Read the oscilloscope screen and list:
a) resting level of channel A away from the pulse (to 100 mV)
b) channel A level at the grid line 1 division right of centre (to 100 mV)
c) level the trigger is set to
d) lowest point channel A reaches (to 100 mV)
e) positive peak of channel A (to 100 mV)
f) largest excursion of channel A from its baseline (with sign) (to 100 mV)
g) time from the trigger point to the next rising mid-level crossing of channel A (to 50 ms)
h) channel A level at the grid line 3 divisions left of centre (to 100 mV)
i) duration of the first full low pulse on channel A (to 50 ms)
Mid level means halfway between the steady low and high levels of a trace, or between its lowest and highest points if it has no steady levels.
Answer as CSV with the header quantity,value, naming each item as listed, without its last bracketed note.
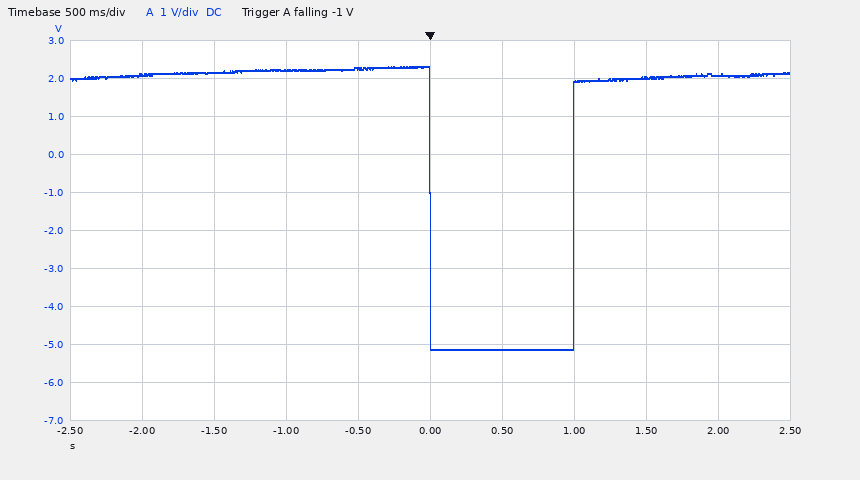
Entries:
quantity,value
resting level of channel A away from the pulse,2.1 V
channel A level at the grid line 1 division right of centre,-5.1 V
level the trigger is set to,-1 V
lowest point channel A reaches,-5.1 V
positive peak of channel A,2.3 V
largest excursion of channel A from its baseline (with sign),-7.2 V
time from the trigger point to the next rising mid-level crossing of channel A,1.00 s
channel A level at the grid line 3 divisions left of centre,2.2 V
duration of the first full low pulse on channel A,1.00 s
